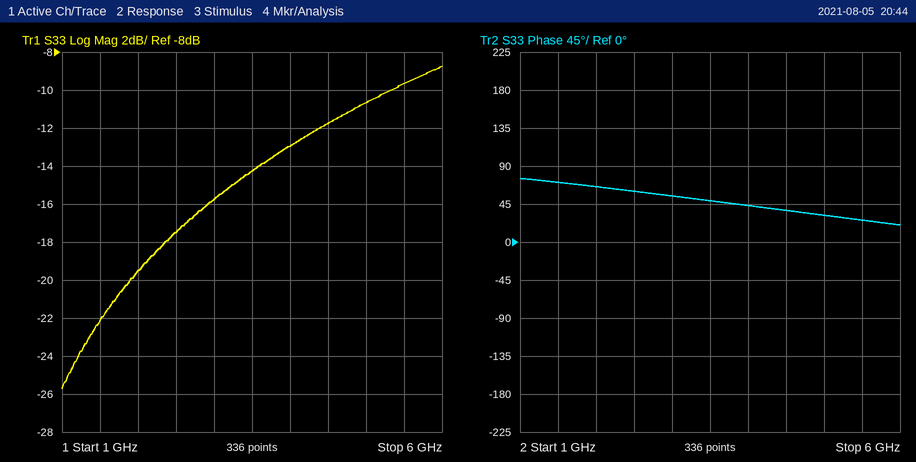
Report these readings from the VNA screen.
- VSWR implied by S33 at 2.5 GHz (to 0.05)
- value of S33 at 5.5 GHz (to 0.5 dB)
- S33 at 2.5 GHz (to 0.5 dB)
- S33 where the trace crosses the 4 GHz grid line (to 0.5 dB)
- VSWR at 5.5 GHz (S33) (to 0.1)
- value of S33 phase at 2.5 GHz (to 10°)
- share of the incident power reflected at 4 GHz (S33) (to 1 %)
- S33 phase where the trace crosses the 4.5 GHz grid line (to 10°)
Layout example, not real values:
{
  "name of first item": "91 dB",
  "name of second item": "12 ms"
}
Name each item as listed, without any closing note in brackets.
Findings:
{
  "VSWR implied by S33 at 2.5 GHz": "1.30",
  "value of S33 at 5.5 GHz": "-9.5 dB",
  "S33 at 2.5 GHz": "-17.5 dB",
  "S33 where the trace crosses the 4 GHz grid line": "-13.0 dB",
  "VSWR at 5.5 GHz (S33)": "2.0",
  "value of S33 phase at 2.5 GHz": "60°",
  "share of the incident power reflected at 4 GHz (S33)": "5 %",
  "S33 phase where the trace crosses the 4.5 GHz grid line": "40°"
}
